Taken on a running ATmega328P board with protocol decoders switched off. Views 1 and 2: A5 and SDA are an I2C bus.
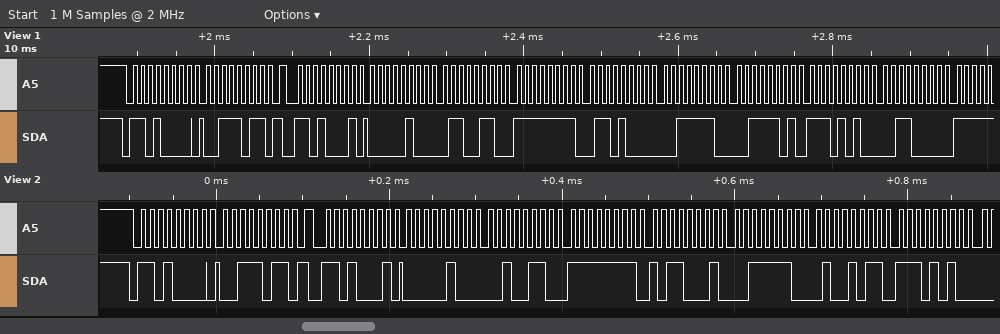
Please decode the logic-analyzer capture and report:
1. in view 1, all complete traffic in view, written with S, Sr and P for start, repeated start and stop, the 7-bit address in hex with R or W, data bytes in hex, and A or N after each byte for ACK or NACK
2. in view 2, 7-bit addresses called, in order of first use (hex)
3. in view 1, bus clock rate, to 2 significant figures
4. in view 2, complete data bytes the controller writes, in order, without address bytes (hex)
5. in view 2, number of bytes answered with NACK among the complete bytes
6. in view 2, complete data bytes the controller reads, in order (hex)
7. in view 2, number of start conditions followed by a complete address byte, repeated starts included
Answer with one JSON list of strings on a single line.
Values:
["S 68W A 3B A Sr 68R A 04 A 66 A FF A 68 A 3E A 3D A EA A 30 A", "0x68", "100 kHz", "3B", "0", "04 26 FF B1 3E 4B EA", "2"]
